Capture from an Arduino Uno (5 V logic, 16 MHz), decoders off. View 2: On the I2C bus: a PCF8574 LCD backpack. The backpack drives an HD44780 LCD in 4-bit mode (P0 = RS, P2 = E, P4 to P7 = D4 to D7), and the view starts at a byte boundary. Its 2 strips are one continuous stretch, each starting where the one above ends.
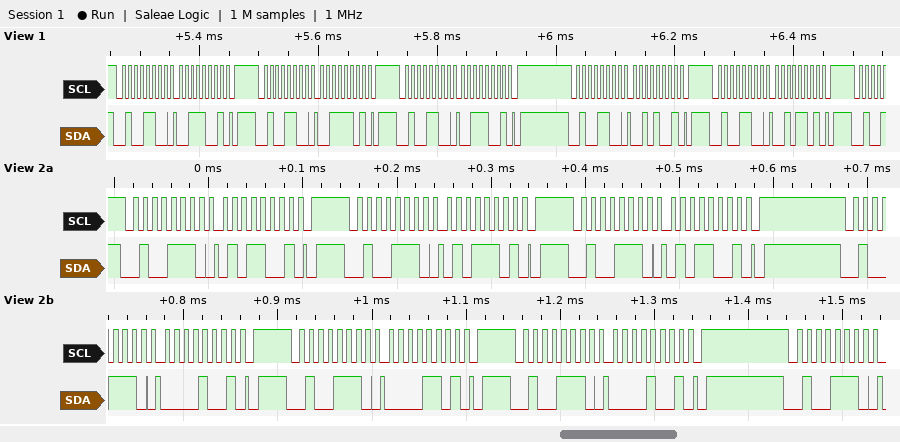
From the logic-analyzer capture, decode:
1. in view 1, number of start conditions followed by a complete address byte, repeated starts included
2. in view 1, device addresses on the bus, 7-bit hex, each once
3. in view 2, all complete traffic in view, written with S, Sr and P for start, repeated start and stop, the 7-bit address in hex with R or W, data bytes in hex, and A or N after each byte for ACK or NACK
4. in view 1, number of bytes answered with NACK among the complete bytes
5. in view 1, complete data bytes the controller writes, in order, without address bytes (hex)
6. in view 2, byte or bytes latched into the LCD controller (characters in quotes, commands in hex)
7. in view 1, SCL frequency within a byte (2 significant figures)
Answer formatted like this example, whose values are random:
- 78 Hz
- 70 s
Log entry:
- 5
- 0x26
- S 27W A 59 A P S 27W A 5D A P S 27W A 59 A P S 27W A 09 A P S 27W A 0D A P S 27W A 09 A P S 27W A
- 0
- 39 3D 39 29 2D
- 'P'
- 100 kHz
